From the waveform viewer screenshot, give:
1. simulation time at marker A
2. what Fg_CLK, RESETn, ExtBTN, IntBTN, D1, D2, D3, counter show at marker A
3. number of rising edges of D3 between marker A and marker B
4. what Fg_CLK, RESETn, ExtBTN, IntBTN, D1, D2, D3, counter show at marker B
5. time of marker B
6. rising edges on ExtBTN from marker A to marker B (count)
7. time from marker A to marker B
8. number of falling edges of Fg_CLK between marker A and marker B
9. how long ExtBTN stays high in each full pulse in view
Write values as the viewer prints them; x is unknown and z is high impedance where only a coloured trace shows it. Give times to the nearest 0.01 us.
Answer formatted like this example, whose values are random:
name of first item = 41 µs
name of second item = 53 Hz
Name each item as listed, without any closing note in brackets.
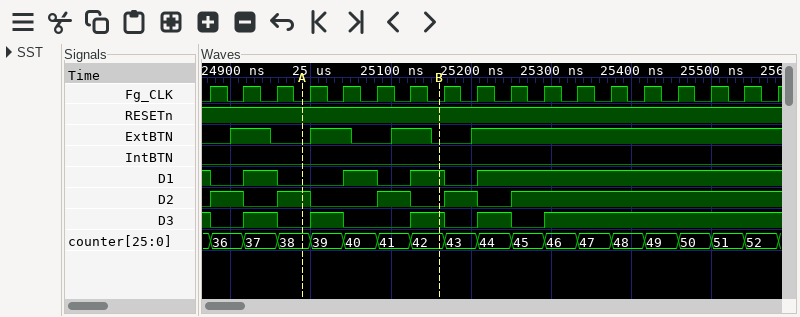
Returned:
simulation time at marker A = 24.99 us
what Fg_CLK, RESETn, ExtBTN, IntBTN, D1, D2, D3, counter show at marker A = Fg_CLK=0, RESETn=1, ExtBTN=0, IntBTN=0, D1=0, D2=1, D3=0, counter=38
number of rising edges of D3 between marker A and marker B = 2
what Fg_CLK, RESETn, ExtBTN, IntBTN, D1, D2, D3, counter show at marker B = Fg_CLK=0, RESETn=1, ExtBTN=0, IntBTN=0, D1=1, D2=0, D3=1, counter=42
time of marker B = 25.16 us
rising edges on ExtBTN from marker A to marker B = 2
time from marker A to marker B = 0.17 us
number of falling edges of Fg_CLK between marker A and marker B = 4
how long ExtBTN stays high in each full pulse in view = 0.05 us, 0.05 us, 0.05 us
